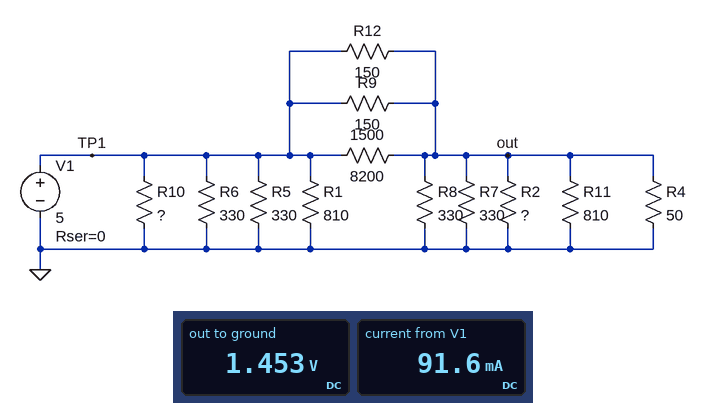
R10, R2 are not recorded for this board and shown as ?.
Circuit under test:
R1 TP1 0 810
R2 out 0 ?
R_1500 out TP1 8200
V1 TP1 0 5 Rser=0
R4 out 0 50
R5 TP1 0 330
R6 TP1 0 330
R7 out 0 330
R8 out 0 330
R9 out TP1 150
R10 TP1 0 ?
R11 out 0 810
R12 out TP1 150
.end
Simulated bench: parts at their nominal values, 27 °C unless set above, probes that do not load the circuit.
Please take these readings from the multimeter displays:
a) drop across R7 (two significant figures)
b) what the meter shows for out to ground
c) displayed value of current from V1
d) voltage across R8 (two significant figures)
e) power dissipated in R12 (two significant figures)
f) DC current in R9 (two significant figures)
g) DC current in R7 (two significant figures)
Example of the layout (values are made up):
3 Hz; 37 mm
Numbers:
1.5 V; 1.453 V; 91.6 mA; 1.5 V; 84 mW; 24 mA; 4.4 mA
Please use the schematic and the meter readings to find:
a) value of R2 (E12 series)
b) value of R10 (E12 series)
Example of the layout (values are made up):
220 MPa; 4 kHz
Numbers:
180 Ω; 680 Ω
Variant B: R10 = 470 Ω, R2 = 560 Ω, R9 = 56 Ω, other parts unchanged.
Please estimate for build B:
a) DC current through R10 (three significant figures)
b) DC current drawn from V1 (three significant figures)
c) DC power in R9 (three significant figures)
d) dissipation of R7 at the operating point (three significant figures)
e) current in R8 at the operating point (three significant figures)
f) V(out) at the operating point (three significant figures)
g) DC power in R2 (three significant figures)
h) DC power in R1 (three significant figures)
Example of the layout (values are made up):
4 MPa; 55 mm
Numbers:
10.6 mA; 114 mA; 131 mW; 15.9 mW; 6.95 mA; 2.29 V; 9.39 mW; 30.9 mW
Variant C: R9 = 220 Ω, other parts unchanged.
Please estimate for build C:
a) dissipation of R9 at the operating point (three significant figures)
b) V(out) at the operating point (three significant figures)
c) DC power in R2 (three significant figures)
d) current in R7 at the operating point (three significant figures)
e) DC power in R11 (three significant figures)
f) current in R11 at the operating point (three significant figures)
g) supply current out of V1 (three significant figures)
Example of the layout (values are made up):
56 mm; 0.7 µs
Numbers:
62.8 mW; 1.28 V; 9.14 mW; 3.89 mA; 2.03 mW; 1.58 mA; 86.0 mA
